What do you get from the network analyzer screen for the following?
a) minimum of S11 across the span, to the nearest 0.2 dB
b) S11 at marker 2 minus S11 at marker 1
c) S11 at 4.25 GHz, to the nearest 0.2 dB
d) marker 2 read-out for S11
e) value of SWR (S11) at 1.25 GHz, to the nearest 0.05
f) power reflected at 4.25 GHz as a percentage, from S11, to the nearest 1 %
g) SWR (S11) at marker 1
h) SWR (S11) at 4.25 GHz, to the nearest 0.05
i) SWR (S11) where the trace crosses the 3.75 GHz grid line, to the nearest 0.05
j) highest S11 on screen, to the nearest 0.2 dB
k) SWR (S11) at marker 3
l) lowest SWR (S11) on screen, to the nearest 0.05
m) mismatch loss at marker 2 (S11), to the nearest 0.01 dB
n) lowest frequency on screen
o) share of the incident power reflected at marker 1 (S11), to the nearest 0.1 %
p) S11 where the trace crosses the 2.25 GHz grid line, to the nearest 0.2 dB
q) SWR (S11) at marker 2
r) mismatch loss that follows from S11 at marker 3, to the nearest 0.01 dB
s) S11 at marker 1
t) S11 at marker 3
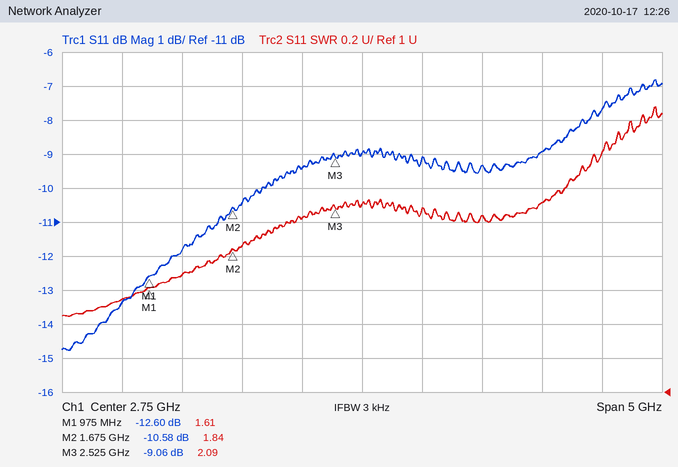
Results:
-14.8 dB
2.02 dB
-9.0 dB
-10.58 dB
1.70
13 %
1.61
2.10
2.05
-6.8 dB
2.09
1.45
0.40 dB
250 MHz
5.5 %
-9.4 dB
1.84
0.58 dB
-12.60 dB
-9.06 dB
